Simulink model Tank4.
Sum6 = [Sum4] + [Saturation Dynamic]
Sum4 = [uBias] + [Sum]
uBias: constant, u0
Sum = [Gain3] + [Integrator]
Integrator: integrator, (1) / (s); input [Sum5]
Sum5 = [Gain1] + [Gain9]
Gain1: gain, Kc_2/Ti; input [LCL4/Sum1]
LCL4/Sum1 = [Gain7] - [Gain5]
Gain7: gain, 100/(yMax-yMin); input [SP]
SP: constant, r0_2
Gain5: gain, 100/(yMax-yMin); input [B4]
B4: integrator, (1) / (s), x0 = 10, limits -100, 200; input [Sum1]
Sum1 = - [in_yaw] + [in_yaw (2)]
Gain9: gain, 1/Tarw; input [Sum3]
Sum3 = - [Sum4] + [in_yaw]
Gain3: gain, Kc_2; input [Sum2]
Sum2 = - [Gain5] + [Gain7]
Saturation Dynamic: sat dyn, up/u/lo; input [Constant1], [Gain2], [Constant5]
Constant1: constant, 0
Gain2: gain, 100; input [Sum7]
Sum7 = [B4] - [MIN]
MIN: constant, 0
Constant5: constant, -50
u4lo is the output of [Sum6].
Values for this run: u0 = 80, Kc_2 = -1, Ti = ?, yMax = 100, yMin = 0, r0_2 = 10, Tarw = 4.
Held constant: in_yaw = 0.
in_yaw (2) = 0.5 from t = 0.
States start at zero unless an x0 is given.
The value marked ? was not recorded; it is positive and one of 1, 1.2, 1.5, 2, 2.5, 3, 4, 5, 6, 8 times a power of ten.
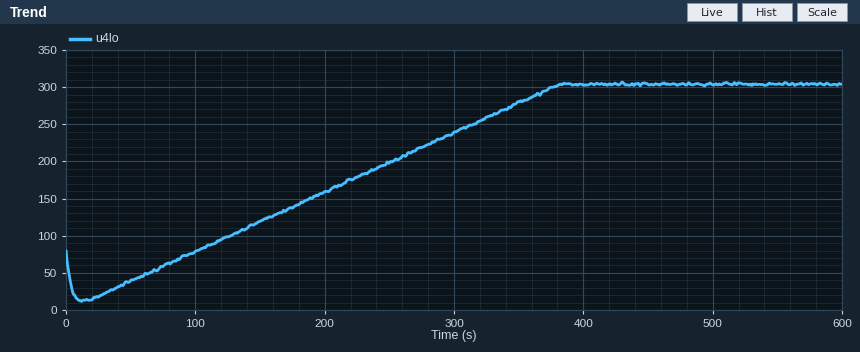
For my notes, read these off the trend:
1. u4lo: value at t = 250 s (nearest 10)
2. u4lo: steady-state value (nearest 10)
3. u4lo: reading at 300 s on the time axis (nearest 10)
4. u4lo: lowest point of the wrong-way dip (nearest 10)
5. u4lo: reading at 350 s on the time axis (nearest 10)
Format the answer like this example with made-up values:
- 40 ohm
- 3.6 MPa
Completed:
- 200
- 300
- 240
- 10
- 280
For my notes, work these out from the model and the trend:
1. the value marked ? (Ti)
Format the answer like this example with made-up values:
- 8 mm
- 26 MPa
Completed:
- 2.5
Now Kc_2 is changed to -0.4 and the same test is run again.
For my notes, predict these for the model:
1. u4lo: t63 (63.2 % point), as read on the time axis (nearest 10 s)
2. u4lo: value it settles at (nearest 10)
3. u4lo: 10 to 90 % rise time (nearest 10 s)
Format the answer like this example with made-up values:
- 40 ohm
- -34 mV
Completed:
- 330 s
- 120
- 100 s
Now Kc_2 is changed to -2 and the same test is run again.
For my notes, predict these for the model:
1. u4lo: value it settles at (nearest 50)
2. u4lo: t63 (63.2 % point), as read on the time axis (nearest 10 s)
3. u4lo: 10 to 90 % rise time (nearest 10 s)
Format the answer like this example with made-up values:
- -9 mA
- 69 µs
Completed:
- 600
- 260 s
- 260 s
